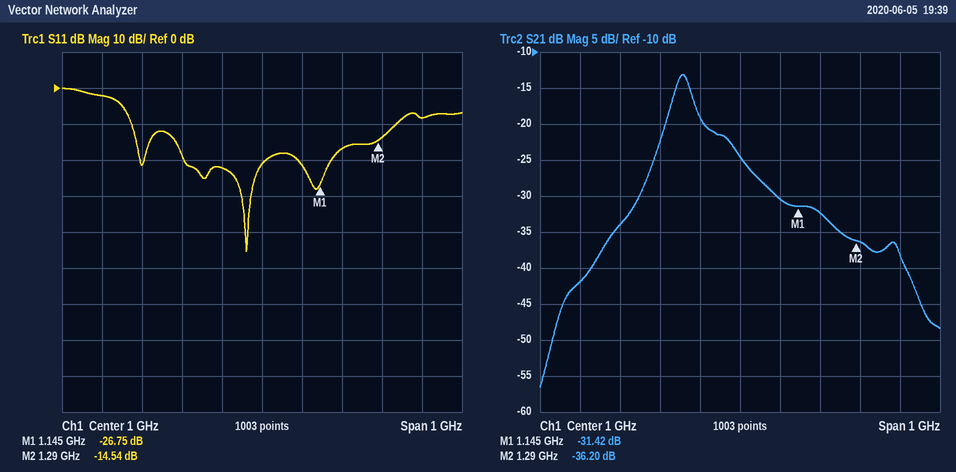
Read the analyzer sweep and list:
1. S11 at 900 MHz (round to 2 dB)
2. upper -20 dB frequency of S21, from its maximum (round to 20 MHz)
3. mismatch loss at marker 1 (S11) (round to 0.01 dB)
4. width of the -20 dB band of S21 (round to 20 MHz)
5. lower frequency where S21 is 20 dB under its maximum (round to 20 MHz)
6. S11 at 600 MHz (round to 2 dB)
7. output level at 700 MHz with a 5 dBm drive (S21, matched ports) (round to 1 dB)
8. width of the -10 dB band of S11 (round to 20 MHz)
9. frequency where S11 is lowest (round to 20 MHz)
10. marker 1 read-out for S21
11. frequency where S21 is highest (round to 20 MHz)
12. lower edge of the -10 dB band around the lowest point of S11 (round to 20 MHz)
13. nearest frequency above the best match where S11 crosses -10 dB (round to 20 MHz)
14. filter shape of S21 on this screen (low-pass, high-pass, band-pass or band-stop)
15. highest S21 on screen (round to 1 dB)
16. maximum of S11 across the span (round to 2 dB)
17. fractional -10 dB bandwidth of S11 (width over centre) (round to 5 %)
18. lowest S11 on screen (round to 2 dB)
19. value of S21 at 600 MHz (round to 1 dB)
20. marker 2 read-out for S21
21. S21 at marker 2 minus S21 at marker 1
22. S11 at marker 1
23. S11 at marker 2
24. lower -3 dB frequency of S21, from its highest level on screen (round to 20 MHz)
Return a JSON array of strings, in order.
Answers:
["-22 dB", "1.22 GHz", "0.01 dB", "500 MHz", "720 MHz", "-2 dB", "-29 dBm", "660 MHz", "960 MHz", "-31.42 dB", "860 MHz", "680 MHz", "1.34 GHz", "band-pass", "-13 dB", "0 dB", "65 %", "-46 dB", "-42 dB", "-36.20 dB", "-4.78 dB", "-26.75 dB", "-14.54 dB", "840 MHz"]
